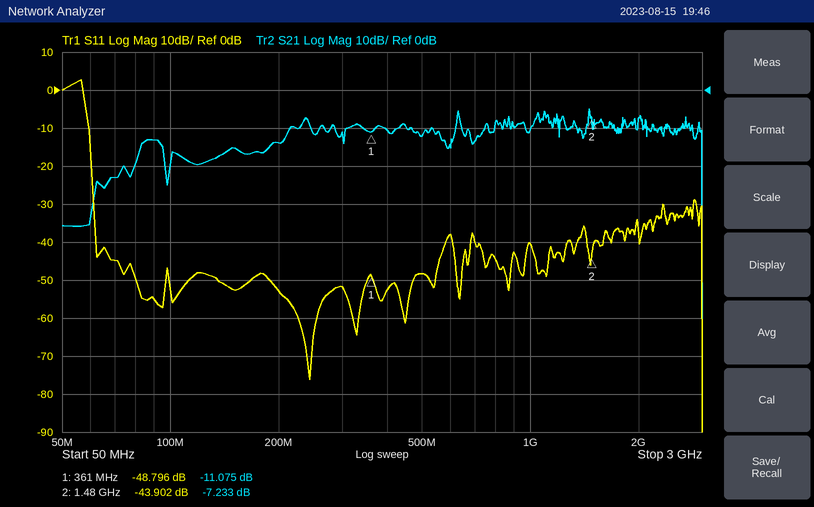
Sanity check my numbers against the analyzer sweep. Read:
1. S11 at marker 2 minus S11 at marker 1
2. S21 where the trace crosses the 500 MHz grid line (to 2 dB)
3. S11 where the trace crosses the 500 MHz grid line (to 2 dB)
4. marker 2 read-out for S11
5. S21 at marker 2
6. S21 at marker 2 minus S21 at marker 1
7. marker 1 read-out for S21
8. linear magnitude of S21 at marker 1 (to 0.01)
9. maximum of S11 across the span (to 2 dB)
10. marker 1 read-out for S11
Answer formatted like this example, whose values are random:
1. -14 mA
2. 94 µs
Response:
1. 4.894 dB
2. -12 dB
3. -48 dB
4. -43.902 dB
5. -7.233 dB
6. 3.842 dB
7. -11.075 dB
8. 0.28
9. 2 dB
10. -48.796 dB
